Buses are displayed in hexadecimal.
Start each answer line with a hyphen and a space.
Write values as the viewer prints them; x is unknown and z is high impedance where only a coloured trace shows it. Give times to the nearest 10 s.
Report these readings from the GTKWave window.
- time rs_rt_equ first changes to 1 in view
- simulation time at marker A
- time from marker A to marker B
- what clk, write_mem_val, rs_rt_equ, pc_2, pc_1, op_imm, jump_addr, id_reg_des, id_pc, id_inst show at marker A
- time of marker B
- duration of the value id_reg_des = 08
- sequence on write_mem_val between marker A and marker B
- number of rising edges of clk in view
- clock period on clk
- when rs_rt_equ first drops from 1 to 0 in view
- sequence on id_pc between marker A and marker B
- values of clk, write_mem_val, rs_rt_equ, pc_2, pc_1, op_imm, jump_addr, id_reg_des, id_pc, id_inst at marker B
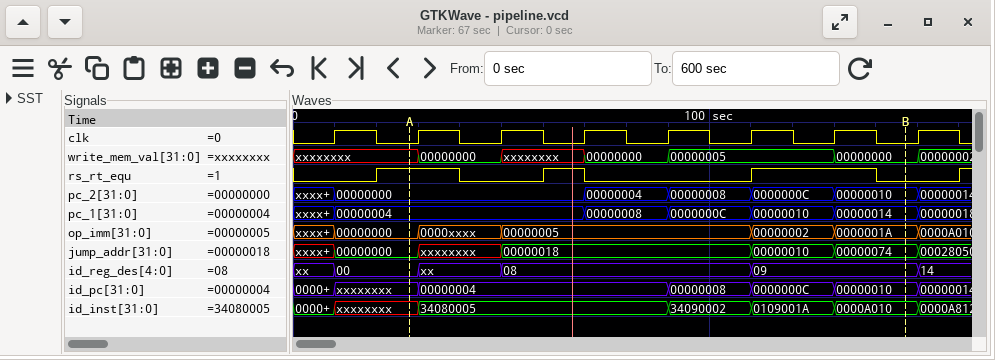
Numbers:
- 20 s
- 30 s
- 120 s
- clk=0, write_mem_val=xxxxxxxx, rs_rt_equ=1, pc_2=00000000, pc_1=00000004, op_imm=00000000, jump_addr=00000000, id_reg_des=00, id_pc=xxxxxxxx, id_inst=xxxxxxxx
- 150 s
- 60 s
- xxxxxxxx, 00000000, xxxxxxxx, 00000000, 00000005, 00000000
- 8
- 20 s
- 40 s
- xxxxxxxx, 00000004, 00000008, 0000000C, 00000010
- clk=0, write_mem_val=00000000, rs_rt_equ=0, pc_2=00000010, pc_1=00000014, op_imm=0000001A, jump_addr=00000074, id_reg_des=09, id_pc=00000010, id_inst=0000A010
